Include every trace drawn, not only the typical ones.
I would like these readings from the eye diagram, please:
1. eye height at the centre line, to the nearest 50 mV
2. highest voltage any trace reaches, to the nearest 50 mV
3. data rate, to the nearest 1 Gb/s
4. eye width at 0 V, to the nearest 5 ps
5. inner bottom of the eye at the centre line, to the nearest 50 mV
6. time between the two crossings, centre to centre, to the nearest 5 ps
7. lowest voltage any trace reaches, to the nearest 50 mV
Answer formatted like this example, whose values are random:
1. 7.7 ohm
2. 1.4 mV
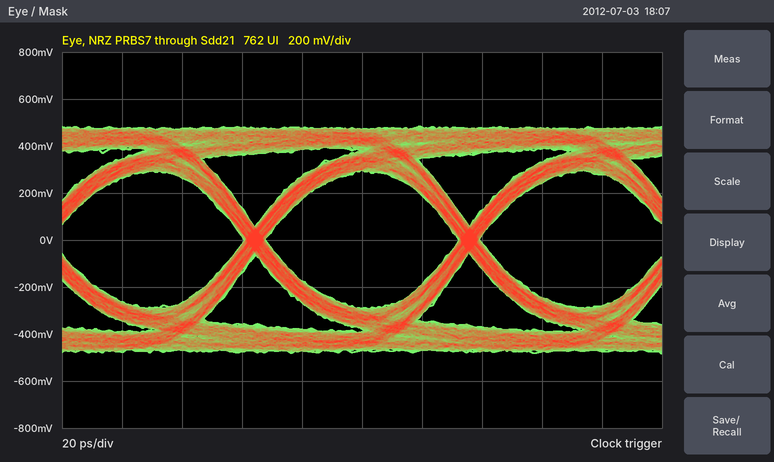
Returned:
1. 600 mV
2. 500 mV
3. 14 Gb/s
4. 65 ps
5. -300 mV
6. 70 ps
7. -500 mV
